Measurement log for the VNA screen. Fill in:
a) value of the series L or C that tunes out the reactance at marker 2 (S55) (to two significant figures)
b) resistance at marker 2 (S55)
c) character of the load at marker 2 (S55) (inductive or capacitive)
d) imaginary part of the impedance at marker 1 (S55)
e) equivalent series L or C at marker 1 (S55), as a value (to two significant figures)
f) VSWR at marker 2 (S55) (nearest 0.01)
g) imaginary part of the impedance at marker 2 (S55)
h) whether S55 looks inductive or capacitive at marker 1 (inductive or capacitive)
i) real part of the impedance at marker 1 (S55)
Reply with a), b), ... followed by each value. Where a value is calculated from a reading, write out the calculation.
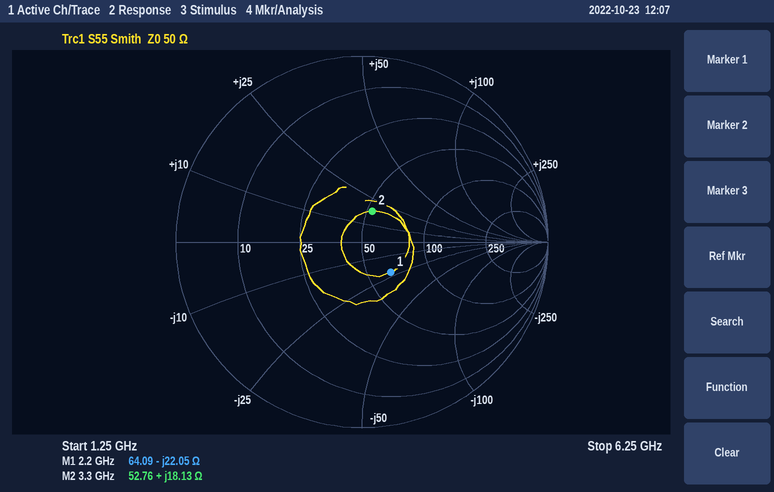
a) C = 1/(2π × 3.3 GHz × 18.13 Ω) ≈ 2.7 pF
b) 52.76 Ω
c) inductive
d) -22.05 Ω
e) C = 1/(2π × 2.2 GHz × 22.05 Ω) ≈ 3.3 pF
f) 1.43
g) +18.13 Ω
h) capacitive
i) 64.09 Ω
